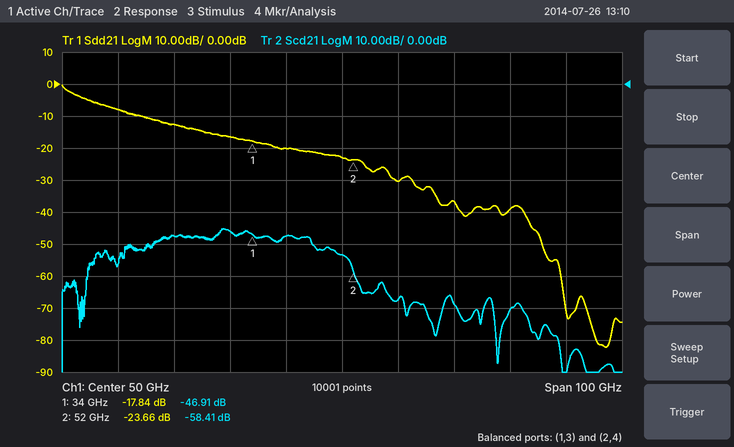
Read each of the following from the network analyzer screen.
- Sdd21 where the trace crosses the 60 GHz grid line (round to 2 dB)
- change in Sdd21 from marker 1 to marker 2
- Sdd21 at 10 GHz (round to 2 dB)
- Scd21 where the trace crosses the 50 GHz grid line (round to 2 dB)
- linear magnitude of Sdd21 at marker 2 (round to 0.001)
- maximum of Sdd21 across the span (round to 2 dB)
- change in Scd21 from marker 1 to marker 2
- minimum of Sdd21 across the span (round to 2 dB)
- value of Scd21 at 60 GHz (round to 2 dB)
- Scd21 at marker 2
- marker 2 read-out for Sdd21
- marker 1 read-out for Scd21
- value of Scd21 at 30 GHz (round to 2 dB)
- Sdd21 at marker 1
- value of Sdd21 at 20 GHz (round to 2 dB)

-30 dB
-5.82 dB
-8 dB
-54 dB
0.066
0 dB
-11.50 dB
-82 dB
-68 dB
-58.41 dB
-23.66 dB
-46.91 dB
-46 dB
-17.84 dB
-12 dB
